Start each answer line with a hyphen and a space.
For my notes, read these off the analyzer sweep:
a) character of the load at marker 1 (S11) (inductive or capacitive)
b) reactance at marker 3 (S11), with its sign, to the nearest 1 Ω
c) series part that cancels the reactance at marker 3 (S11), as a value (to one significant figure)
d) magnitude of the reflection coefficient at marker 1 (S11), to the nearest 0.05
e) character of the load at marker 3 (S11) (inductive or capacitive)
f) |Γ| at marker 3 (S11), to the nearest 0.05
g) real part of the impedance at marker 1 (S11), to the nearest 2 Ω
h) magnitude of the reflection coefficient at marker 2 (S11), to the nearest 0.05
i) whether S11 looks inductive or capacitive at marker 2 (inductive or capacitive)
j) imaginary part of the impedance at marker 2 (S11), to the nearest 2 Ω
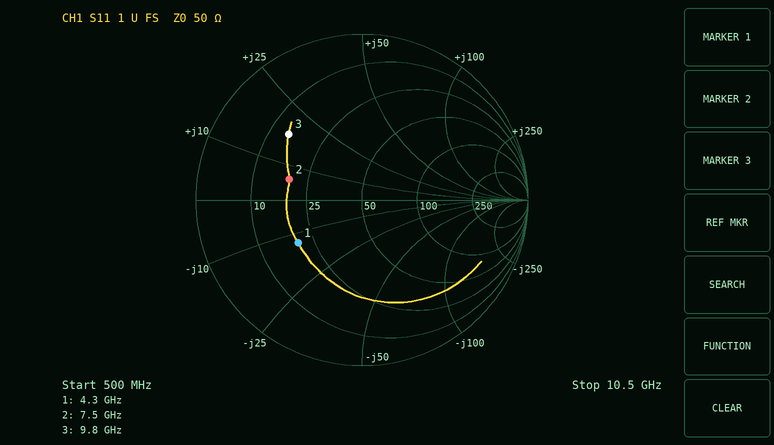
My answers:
- capacitive
- +18 Ω
- 900 fF
- 0.45
- inductive
- 0.60
- 20 Ω
- 0.45
- inductive
- +6 Ω
